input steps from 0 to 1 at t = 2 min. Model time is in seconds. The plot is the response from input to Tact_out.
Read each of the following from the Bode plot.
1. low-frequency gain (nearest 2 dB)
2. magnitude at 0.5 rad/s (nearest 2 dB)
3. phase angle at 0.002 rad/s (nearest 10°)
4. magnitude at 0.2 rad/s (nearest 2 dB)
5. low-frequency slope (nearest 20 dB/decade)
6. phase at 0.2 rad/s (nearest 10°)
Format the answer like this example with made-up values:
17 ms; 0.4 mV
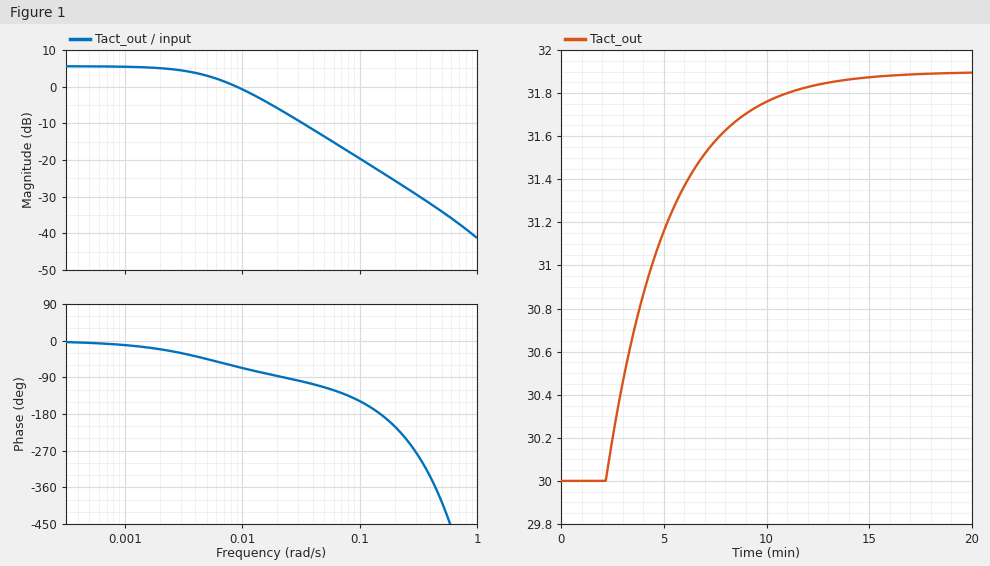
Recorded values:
6 dB; -34 dB; -20°; -26 dB; 0 dB/decade; -210°
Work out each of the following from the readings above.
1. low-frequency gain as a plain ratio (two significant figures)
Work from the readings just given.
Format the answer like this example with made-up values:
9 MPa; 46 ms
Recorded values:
2.0
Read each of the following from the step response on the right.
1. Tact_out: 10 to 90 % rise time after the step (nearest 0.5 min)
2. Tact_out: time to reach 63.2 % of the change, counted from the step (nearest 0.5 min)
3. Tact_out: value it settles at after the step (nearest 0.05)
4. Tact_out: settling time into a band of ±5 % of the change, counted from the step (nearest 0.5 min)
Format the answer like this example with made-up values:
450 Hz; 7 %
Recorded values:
6.5 min; 3.0 min; 31.90; 9.0 min
